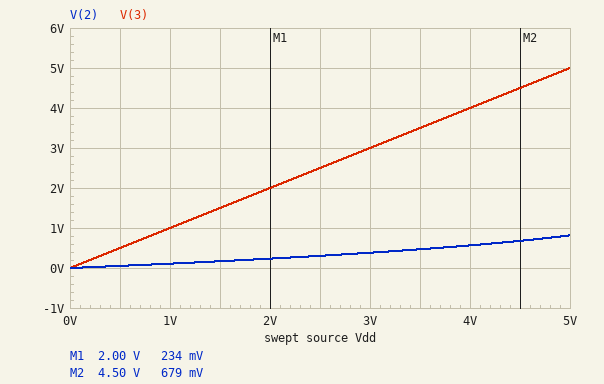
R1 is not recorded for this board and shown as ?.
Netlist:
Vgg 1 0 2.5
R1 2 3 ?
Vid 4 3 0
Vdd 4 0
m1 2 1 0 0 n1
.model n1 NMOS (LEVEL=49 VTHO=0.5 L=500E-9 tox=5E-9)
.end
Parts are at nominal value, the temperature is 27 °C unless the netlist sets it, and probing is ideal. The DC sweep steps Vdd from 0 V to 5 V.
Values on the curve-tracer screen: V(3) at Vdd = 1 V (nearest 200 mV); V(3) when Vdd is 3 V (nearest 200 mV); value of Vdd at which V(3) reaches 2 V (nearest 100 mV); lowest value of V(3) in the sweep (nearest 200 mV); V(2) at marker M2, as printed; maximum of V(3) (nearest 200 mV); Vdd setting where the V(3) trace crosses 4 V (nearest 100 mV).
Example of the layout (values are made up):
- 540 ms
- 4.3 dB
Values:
- 1.0 V
- 3.0 V
- 2.0 V
- 0 V
- 679 mV
- 5.0 V
- 4.0 V
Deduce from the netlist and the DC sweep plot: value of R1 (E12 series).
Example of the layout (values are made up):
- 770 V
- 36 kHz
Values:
- 2.7 kΩ
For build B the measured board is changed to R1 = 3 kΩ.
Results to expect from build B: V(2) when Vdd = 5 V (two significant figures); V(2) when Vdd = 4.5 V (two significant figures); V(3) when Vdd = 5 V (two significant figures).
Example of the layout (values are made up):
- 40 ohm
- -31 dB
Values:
- 700 mV
- 590 mV
- 5.0 V
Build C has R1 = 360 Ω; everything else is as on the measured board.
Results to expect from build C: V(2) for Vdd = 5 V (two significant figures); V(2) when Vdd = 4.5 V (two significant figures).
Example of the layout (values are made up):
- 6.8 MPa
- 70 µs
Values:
- 4.2 V
- 3.8 V
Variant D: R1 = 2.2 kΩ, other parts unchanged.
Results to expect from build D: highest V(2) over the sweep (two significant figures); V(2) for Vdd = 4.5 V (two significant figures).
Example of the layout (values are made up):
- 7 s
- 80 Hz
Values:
- 1.2 V
- 920 mV
